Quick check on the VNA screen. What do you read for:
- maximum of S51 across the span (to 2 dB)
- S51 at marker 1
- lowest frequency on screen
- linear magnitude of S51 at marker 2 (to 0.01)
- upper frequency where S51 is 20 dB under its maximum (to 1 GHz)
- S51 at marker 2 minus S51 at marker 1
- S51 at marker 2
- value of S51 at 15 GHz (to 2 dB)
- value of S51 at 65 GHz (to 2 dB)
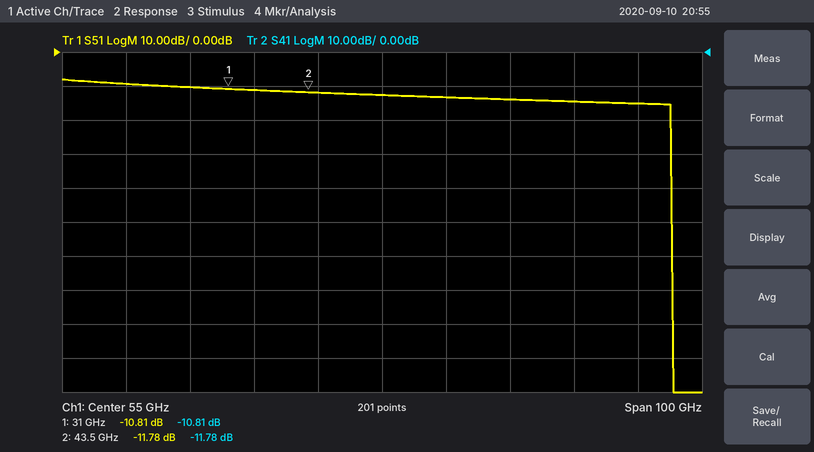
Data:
-8 dB
-10.81 dB
5 GHz
0.26
100 GHz
-0.97 dB
-11.78 dB
-10 dB
-14 dB
